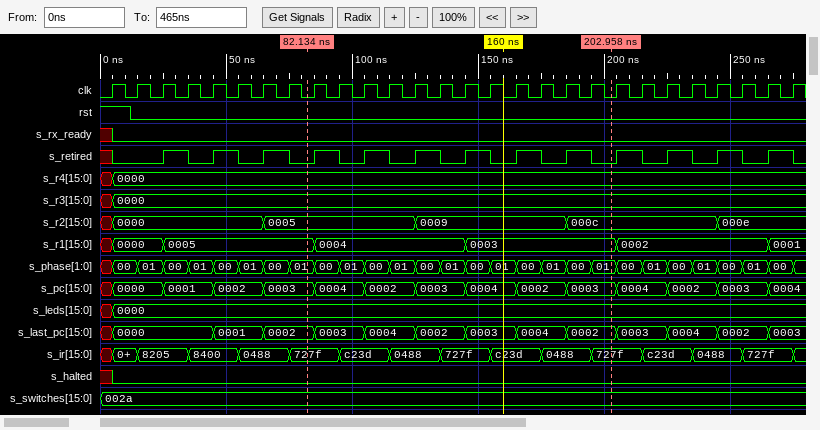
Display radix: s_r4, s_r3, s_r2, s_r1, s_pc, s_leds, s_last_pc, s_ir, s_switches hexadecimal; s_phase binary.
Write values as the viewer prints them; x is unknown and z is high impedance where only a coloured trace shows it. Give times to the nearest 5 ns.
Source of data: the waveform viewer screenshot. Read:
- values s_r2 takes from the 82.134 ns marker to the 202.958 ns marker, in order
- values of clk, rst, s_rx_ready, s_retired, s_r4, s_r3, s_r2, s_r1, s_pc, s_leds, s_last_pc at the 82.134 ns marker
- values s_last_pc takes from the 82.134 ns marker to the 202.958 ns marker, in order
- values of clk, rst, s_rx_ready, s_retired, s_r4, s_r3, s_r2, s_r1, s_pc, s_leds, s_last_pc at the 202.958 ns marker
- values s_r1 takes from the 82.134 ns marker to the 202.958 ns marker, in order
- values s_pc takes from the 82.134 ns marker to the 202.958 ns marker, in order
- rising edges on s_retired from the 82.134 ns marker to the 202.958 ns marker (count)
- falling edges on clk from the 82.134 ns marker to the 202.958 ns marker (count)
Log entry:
0005, 0009, 000c
clk=0, rst=0, s_rx_ready=0, s_retired=0, s_r4=0000, s_r3=0000, s_r2=0005, s_r1=0005, s_pc=0003, s_leds=0000, s_last_pc=0002
0002, 0003, 0004, 0002, 0003, 0004, 0002
clk=0, rst=0, s_rx_ready=0, s_retired=0, s_r4=0000, s_r3=0000, s_r2=000c, s_r1=0003, s_pc=0003, s_leds=0000, s_last_pc=0002
0005, 0004, 0003
0003, 0004, 0002, 0003, 0004, 0002, 0003
6
12
